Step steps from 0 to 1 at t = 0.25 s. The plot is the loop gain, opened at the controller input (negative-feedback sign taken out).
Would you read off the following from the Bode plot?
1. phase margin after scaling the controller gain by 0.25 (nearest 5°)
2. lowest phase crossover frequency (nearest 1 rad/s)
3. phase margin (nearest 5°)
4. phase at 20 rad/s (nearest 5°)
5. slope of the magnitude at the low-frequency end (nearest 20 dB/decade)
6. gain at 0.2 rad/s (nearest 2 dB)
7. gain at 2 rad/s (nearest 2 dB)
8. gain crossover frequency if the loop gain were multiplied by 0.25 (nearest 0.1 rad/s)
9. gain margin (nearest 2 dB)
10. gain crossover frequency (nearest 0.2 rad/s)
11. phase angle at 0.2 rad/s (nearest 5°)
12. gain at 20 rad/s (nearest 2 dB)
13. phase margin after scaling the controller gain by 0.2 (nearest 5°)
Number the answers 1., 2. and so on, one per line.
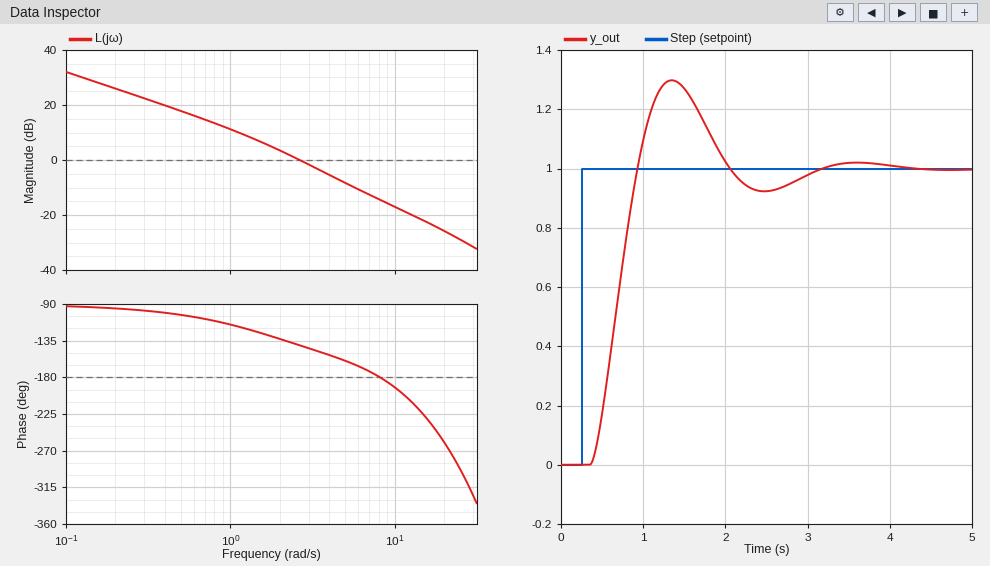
1. 65°
2. 8 rad/s
3. 40°
4. -260°
5. -20 dB/decade
6. 26 dB
7. 4 dB
8. 0.9 rad/s
9. 14 dB
10. 2.6 rad/s
11. -95°
12. -26 dB
13. 70°
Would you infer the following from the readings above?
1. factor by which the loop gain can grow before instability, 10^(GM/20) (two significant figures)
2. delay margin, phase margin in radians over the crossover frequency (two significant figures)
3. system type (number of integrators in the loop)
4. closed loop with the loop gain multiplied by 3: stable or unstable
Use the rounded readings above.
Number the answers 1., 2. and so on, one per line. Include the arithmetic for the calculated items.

1. 10^(14 / 20) = 5.0
2. 40 × π / 180 / 2.6 = 0.27 s
3. 1
4. stable
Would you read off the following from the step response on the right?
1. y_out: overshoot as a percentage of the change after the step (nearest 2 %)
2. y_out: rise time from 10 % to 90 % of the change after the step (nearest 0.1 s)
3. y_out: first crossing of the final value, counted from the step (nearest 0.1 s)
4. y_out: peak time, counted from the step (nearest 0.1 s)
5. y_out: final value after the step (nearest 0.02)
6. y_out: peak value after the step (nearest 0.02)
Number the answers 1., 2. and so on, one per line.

1. 30 %
2. 0.4 s
3. 0.7 s
4. 1.1 s
5. 1.00
6. 1.30
